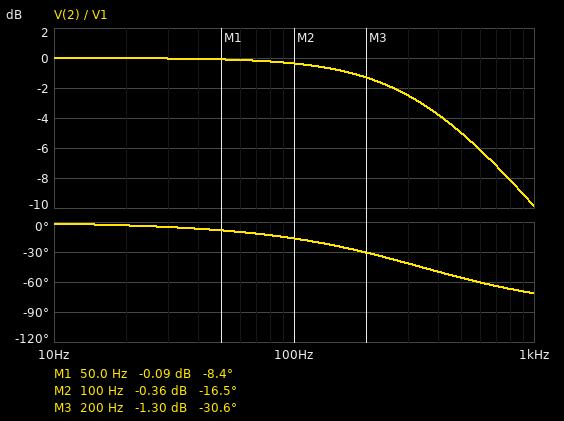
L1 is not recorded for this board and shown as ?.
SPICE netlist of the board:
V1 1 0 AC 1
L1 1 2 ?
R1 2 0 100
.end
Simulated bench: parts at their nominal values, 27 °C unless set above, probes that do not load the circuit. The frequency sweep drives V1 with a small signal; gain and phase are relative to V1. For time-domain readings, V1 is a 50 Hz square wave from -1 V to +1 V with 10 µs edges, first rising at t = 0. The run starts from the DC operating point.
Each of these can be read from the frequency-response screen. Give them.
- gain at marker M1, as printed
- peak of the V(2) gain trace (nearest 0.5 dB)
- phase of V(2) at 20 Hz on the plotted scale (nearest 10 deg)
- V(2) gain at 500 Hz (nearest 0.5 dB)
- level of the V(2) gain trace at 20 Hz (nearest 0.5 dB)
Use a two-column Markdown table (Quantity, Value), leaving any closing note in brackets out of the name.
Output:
| Quantity | Value |
|---|---|
| gain at marker M1, as printed | -0.09 dB |
| peak of the V(2) gain trace | 0 dB |
| phase of V(2) at 20 Hz on the plotted scale | 0 deg |
| V(2) gain at 500 Hz | -5.0 dB |
| level of the V(2) gain trace at 20 Hz | 0 dB |
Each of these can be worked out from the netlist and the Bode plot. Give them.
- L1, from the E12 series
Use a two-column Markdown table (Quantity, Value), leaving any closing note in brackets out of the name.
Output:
| Quantity | Value |
|---|---|
| L1, from the E12 series | 47 mH |
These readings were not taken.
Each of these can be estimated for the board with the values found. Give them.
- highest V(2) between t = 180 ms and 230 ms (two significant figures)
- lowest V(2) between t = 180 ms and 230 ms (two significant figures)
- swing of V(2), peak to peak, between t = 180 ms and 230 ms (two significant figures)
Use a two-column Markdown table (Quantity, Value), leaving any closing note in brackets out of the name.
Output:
| Quantity | Value |
|---|---|
| highest V(2) between t = 180 ms and 230 ms | 1.0 V |
| lowest V(2) between t = 180 ms and 230 ms | -1.0 V |
| swing of V(2), peak to peak, between t = 180 ms and 230 ms | 2.0 V |
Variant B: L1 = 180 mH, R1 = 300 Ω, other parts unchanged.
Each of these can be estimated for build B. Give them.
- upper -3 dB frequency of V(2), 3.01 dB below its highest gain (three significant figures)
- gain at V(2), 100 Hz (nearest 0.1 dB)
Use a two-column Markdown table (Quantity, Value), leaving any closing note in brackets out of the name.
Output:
| Quantity | Value |
|---|---|
| upper -3 dB frequency of V(2), 3.01 dB below its highest gain | 265 Hz |
| gain at V(2), 100 Hz | -0.6 dB |
